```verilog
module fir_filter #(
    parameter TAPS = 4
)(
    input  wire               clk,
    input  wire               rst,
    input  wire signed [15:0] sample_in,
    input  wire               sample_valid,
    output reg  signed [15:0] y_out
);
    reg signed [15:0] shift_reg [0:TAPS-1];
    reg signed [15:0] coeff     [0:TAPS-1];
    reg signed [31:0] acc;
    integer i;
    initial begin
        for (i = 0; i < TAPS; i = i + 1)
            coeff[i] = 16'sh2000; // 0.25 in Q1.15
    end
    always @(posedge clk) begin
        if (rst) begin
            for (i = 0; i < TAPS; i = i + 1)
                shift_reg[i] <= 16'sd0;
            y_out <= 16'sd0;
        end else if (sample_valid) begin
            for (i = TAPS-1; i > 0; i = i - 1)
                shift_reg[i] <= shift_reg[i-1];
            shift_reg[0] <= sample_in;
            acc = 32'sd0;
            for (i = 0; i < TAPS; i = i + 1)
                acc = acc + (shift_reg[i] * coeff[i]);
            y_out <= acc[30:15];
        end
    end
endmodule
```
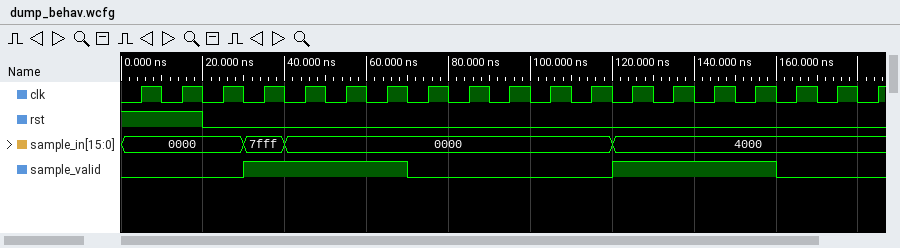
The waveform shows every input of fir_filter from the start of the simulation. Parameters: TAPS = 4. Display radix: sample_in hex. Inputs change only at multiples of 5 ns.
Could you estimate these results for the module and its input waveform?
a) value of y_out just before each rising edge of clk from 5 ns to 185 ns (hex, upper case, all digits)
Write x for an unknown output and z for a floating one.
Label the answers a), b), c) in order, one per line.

a) x, 0000, 0000, 0000, 0000, 1FFF, 1FFF, 1FFF, 1FFF, 1FFF, 1FFF, 1FFF, 1FFF, 1FFF, 1000, 2000, 3000, 3000, 3000
